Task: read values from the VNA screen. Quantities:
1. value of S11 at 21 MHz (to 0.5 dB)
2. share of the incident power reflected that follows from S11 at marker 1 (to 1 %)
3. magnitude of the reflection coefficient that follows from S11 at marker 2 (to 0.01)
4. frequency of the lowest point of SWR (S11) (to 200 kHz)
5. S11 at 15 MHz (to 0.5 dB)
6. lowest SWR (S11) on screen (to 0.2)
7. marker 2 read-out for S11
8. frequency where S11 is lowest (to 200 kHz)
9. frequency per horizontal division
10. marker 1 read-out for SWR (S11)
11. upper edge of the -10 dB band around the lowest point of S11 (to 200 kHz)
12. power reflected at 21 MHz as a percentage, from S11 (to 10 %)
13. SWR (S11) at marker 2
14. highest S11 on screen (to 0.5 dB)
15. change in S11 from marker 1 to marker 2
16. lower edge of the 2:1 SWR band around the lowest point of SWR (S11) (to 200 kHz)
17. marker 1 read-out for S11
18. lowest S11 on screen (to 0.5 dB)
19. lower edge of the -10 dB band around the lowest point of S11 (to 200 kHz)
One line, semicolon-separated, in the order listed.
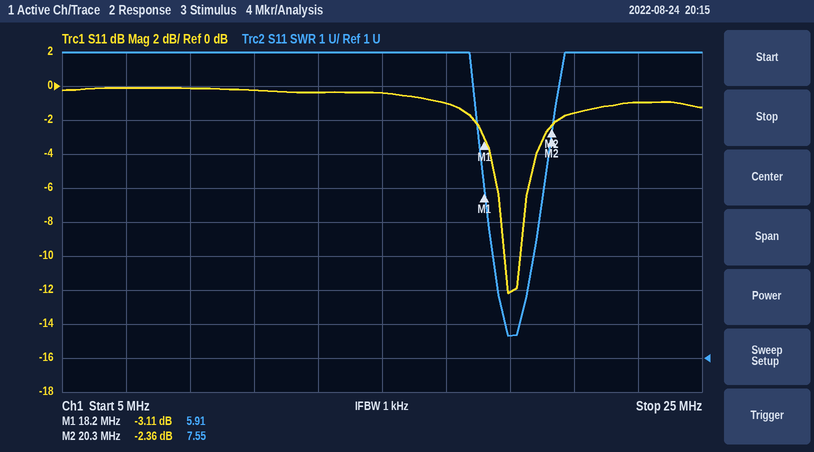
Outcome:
-1.5 dB; 49 %; 0.76; 19.0 MHz; -0.5 dB; 1.6; -2.36 dB; 19.0 MHz; 2 MHz; 5.91; 19.4 MHz; 70 %; 7.55; 0.0 dB; 0.75 dB; 18.8 MHz; -3.11 dB; -12.0 dB; 18.8 MHz
